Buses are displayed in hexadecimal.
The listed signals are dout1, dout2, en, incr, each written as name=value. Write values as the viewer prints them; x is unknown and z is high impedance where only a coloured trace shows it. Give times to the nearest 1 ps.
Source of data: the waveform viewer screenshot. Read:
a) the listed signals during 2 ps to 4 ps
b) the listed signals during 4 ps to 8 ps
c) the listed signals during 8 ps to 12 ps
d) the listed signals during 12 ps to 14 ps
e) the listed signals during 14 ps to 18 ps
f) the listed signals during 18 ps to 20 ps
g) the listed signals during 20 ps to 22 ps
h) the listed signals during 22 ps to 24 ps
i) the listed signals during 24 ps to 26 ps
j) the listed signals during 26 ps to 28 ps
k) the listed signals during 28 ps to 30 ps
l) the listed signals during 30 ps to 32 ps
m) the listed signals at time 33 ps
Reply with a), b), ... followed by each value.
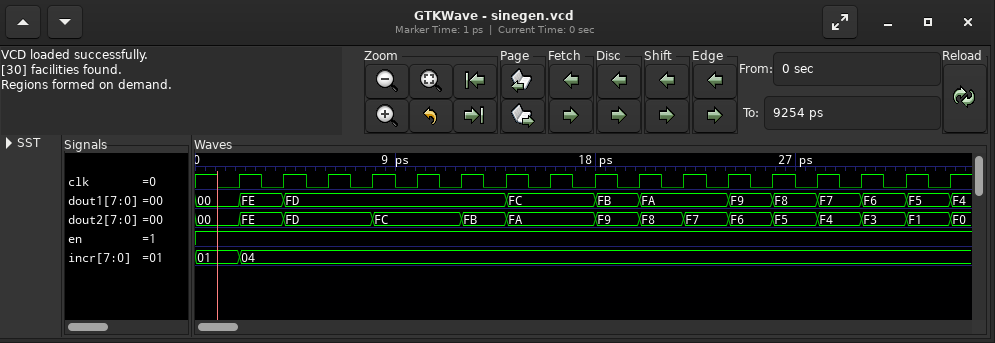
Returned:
a) dout1=FE, dout2=FE, en=1, incr=04
b) dout1=FD, dout2=FD, en=1, incr=04
c) dout1=FD, dout2=FC, en=1, incr=04
d) dout1=FD, dout2=FB, en=1, incr=04
e) dout1=FC, dout2=FA, en=1, incr=04
f) dout1=FB, dout2=F9, en=1, incr=04
g) dout1=FA, dout2=F8, en=1, incr=04
h) dout1=FA, dout2=F7, en=1, incr=04
i) dout1=F9, dout2=F6, en=1, incr=04
j) dout1=F8, dout2=F5, en=1, incr=04
k) dout1=F7, dout2=F4, en=1, incr=04
l) dout1=F6, dout2=F3, en=1, incr=04
m) dout1=F5, dout2=F1, en=1, incr=04
